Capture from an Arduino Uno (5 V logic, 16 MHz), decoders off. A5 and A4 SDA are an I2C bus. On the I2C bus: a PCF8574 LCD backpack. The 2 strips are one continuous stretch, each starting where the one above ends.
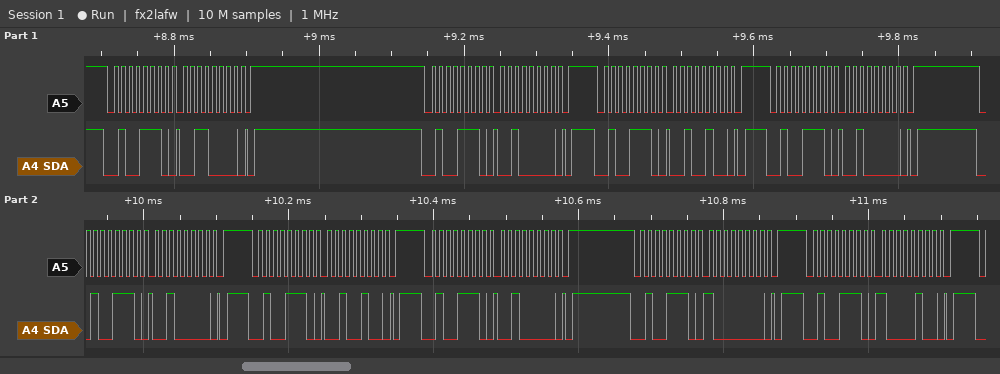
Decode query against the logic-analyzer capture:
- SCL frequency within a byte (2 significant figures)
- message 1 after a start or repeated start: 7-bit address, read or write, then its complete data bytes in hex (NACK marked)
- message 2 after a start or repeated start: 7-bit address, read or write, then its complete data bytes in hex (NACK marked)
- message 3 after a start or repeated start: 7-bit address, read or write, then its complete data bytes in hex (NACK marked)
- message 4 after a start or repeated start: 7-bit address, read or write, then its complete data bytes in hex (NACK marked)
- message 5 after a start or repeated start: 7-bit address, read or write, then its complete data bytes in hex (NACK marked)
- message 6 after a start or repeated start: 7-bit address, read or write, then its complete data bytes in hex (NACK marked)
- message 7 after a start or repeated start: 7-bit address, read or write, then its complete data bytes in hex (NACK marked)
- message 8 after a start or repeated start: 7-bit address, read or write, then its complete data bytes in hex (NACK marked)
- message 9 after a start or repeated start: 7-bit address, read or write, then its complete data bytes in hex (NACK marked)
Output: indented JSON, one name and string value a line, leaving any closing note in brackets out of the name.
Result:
{
  "SCL frequency within a byte": "100 kHz",
  "message 1 after a start or repeated start: 7-bit address, read or write, then its complete data bytes in hex": "0x27 write: 30",
  "message 2 after a start or repeated start: 7-bit address, read or write, then its complete data bytes in hex": "0x27 write: 20",
  "message 3 after a start or repeated start: 7-bit address, read or write, then its complete data bytes in hex": "0x27 write: 24",
  "message 4 after a start or repeated start: 7-bit address, read or write, then its complete data bytes in hex": "0x27 write: 20",
  "message 5 after a start or repeated start: 7-bit address, read or write, then its complete data bytes in hex": "0x27 write: 20",
  "message 6 after a start or repeated start: 7-bit address, read or write, then its complete data bytes in hex": "0x27 write: 24",
  "message 7 after a start or repeated start: 7-bit address, read or write, then its complete data bytes in hex": "0x27 write: 20",
  "message 8 after a start or repeated start: 7-bit address, read or write, then its complete data bytes in hex": "0x27 write: 80",
  "message 9 after a start or repeated start: 7-bit address, read or write, then its complete data bytes in hex": "0x27 write: 84"
}
